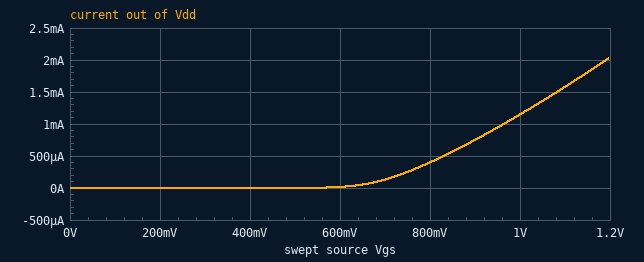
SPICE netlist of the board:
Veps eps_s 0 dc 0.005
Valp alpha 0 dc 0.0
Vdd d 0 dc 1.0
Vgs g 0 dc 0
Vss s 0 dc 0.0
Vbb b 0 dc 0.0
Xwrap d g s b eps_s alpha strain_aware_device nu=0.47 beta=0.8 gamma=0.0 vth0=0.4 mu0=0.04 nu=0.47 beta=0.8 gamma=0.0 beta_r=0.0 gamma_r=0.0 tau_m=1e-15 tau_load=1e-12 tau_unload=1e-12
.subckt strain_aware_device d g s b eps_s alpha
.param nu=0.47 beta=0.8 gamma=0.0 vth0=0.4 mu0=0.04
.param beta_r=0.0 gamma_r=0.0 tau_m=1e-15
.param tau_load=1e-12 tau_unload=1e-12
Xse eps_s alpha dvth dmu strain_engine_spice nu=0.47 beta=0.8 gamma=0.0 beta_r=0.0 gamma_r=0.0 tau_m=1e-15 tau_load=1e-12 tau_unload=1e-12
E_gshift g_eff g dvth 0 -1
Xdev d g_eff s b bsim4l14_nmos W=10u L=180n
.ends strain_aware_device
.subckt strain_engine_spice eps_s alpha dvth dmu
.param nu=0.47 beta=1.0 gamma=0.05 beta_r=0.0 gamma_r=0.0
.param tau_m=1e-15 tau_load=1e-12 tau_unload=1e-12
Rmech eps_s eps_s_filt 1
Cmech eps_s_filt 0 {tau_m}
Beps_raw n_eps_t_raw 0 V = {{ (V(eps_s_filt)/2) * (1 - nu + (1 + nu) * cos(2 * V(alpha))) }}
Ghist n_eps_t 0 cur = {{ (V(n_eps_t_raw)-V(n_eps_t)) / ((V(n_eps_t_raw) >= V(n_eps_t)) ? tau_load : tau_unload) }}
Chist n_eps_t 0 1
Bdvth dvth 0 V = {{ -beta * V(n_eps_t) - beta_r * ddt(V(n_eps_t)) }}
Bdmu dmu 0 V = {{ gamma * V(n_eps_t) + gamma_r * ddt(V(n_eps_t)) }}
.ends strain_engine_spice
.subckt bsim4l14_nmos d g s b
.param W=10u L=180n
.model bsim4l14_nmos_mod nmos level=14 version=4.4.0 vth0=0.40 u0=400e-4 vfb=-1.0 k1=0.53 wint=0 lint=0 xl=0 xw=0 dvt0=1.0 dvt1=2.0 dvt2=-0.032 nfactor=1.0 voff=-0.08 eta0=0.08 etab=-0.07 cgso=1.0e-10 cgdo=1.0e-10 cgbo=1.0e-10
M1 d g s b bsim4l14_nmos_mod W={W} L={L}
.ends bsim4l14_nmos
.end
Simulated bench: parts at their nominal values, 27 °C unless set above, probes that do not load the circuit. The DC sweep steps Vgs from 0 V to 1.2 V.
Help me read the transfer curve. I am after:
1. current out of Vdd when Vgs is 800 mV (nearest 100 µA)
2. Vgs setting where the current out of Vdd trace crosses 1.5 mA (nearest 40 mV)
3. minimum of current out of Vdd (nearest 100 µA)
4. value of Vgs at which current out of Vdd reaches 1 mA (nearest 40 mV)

400 µA
1.08 V
0 A
960 mV
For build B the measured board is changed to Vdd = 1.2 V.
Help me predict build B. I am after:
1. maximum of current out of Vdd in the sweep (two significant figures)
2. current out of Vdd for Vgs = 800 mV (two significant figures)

2.1 mA
420 µA
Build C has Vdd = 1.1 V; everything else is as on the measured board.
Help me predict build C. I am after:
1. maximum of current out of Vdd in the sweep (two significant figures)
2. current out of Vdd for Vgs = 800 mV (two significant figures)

2.1 mA
410 µA
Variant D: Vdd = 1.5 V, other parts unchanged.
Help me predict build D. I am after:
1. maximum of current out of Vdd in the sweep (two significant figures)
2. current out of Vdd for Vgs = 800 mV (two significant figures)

2.2 mA
460 µA
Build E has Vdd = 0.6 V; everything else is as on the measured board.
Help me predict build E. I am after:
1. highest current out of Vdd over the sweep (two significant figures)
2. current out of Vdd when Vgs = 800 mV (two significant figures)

1.8 mA
350 µA
